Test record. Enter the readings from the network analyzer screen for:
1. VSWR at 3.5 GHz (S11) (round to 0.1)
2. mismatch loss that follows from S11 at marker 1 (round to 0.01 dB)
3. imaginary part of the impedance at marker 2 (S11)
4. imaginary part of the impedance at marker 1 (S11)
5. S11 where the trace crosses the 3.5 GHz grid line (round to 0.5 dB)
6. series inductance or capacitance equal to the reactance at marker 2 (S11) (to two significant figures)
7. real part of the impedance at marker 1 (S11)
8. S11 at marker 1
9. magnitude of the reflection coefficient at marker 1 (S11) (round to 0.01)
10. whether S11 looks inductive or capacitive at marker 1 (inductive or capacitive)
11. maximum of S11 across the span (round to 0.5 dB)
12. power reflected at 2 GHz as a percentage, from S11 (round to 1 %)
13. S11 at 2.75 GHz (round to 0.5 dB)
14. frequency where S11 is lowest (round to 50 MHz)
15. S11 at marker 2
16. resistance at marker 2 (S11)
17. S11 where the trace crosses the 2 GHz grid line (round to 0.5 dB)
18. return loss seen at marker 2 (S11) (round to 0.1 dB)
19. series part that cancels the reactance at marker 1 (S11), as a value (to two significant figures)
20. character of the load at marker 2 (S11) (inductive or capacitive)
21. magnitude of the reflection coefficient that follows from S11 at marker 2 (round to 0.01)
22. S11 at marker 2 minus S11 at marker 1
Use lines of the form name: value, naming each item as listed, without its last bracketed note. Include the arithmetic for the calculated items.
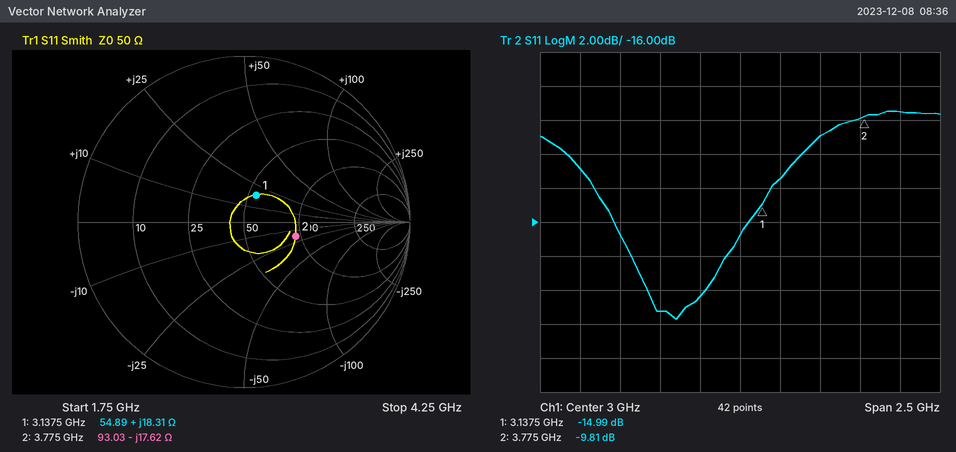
VSWR at 3.5 GHz (S11): |Γ| = 10^(-11/20) = 0.2818; VSWR = (1 + 0.2818)/(1 − 0.2818) ≈ 1.8
mismatch loss that follows from S11 at marker 1: −10 log10(1 − 10^(-14.99/10)) ≈ 0.14 dB
imaginary part of the impedance at marker 2: -17.62 Ω
imaginary part of the impedance at marker 1: +18.31 Ω
S11 where the trace crosses the 3.5 GHz grid line: -11.0 dB
series inductance or capacitance equal to the reactance at marker 2 (S11): C = 1/(2π × 3.775 GHz × 17.62 Ω) ≈ 2.4 pF
real part of the impedance at marker 1: 54.89 Ω
S11 at marker 1: -14.99 dB
magnitude of the reflection coefficient at marker 1 (S11): 0.18
whether S11 looks inductive or capacitive at marker 1: inductive
maximum of S11 across the span: -9.5 dB
power reflected at 2 GHz as a percentage, from S11: 10^(-13/10) ≈ 5 %
S11 at 2.75 GHz: -20.5 dB
frequency where S11 is lowest: 2.60 GHz
S11 at marker 2: -9.81 dB
resistance at marker 2: 93.03 Ω
S11 where the trace crosses the 2 GHz grid line: -13.0 dB
return loss seen at marker 2 (S11): 9.8 dB
series part that cancels the reactance at marker 1 (S11), as a value: C = 1/(2π × 3.1375 GHz × 18.31 Ω) ≈ 2.8 pF
character of the load at marker 2 (S11): capacitive
magnitude of the reflection coefficient that follows from S11 at marker 2: 10^(-9.81/20) ≈ 0.32
S11 at marker 2 minus S11 at marker 1: -9.81 − (-14.99) = 5.18 dB
